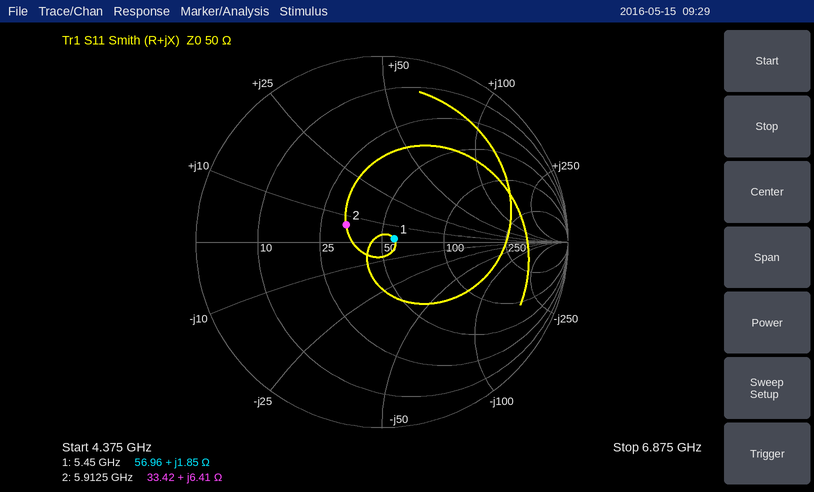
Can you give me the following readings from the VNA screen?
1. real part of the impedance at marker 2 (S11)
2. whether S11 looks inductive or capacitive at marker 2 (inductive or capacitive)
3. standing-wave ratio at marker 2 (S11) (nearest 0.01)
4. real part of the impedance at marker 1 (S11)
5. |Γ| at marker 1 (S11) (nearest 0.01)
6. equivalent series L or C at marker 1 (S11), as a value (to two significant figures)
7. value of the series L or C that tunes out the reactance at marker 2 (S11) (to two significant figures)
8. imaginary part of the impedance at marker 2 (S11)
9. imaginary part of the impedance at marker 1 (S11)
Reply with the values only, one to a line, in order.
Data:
33.42 Ω
inductive
1.54
56.96 Ω
0.07
54 pH
4.2 pF
+6.41 Ω
+1.85 Ω
